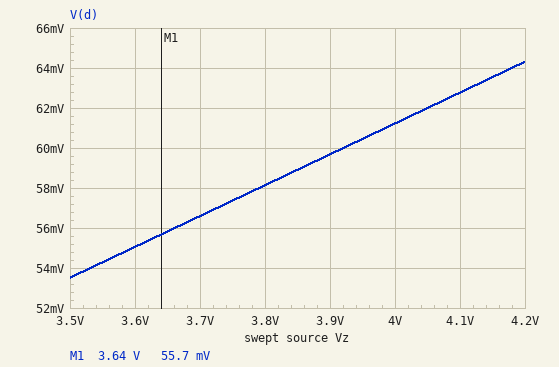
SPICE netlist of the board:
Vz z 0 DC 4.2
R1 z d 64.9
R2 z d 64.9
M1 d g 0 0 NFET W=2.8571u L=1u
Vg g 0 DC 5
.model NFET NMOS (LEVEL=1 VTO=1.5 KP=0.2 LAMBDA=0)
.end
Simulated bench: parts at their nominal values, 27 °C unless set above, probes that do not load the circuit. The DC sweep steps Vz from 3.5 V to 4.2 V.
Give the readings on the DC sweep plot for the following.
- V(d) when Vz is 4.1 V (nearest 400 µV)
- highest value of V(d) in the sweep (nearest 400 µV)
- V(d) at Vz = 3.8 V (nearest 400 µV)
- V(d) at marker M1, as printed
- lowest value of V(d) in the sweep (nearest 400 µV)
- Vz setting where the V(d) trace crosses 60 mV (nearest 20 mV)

62.8 mV
64.4 mV
58.0 mV
55.7 mV
53.6 mV
3.92 V
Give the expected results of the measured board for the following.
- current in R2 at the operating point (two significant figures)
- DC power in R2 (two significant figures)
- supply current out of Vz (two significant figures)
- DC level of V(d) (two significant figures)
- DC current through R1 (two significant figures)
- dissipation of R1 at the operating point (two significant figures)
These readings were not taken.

64 mA
260 mW
130 mA
64 mV
64 mA
260 mW
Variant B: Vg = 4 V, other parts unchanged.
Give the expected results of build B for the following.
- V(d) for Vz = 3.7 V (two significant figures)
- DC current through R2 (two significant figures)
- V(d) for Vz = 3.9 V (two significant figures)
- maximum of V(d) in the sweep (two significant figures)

79 mV
63 mA
84 mV
90 mV
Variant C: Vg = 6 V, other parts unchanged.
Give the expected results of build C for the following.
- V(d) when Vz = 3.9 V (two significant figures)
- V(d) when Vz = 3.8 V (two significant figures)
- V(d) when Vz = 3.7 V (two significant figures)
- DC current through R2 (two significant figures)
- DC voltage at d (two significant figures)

46 mV
45 mV
44 mV
64 mA
50 mV
